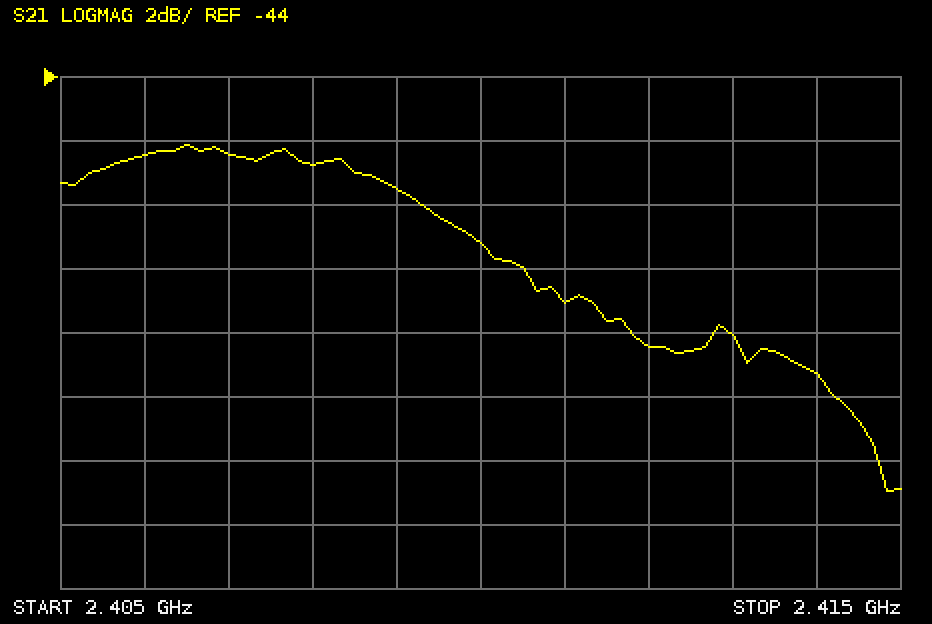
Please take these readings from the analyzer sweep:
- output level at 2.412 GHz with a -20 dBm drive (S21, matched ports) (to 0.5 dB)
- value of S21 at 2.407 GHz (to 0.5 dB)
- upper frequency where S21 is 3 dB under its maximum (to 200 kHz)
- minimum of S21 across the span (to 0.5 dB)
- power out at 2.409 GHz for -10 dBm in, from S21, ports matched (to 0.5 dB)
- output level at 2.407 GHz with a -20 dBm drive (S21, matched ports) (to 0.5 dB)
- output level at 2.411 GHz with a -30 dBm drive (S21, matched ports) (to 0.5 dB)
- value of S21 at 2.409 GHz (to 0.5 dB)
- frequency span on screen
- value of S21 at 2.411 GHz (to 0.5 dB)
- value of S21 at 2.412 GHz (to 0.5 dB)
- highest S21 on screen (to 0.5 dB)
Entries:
-72.5 dBm
-46.5 dB
2.4100 GHz
-57.0 dB
-57.5 dBm
-66.5 dBm
-81.0 dBm
-47.5 dB
10 MHz
-51.0 dB
-52.5 dB
-46.0 dB
